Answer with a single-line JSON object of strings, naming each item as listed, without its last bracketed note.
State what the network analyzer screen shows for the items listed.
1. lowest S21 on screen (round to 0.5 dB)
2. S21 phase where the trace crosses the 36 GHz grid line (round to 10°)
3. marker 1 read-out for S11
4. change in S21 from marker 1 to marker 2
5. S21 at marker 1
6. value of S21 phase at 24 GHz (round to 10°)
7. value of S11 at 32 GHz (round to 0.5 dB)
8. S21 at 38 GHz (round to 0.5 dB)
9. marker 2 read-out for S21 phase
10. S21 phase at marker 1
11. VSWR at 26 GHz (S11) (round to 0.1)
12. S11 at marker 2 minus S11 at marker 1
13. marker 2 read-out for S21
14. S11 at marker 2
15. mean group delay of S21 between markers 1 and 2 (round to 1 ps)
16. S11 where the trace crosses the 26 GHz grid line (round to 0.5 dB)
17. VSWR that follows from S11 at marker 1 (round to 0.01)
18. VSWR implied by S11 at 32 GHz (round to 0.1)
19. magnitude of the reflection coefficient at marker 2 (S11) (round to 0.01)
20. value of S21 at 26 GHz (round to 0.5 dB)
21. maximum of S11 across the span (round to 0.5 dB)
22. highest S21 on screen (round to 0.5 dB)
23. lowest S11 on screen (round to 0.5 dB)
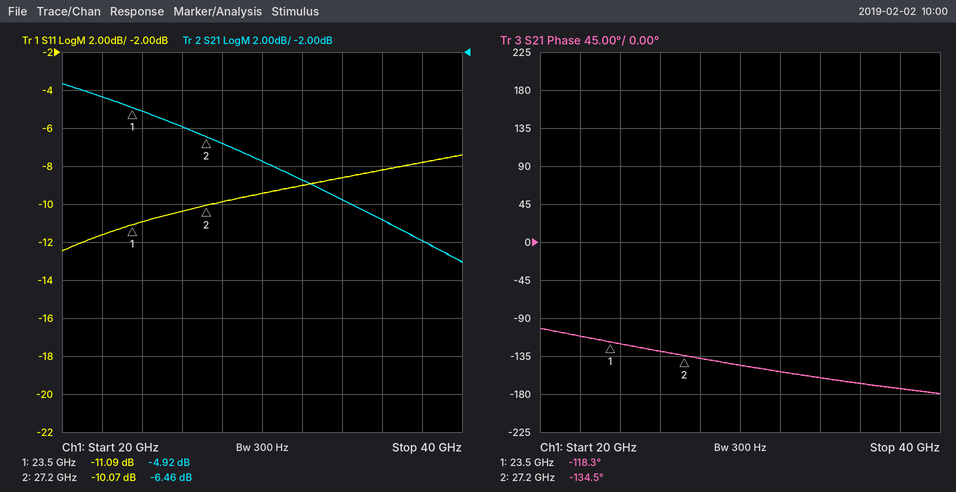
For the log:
{"lowest S21 on screen": "-13.0 dB", "S21 phase where the trace crosses the 36 GHz grid line": "-170°", "marker 1 read-out for S11": "-11.09 dB", "change in S21 from marker 1 to marker 2": "-1.54 dB", "S21 at marker 1": "-4.92 dB", "value of S21 phase at 24 GHz": "-120°", "value of S11 at 32 GHz": "-9.0 dB", "S21 at 38 GHz": "-12.0 dB", "marker 2 read-out for S21 phase": "-134.5°", "S21 phase at marker 1": "-118.3°", "VSWR at 26 GHz (S11)": "1.9", "S11 at marker 2 minus S11 at marker 1": "1.02 dB", "marker 2 read-out for S21": "-6.46 dB", "S11 at marker 2": "-10.07 dB", "mean group delay of S21 between markers 1 and 2": "12 ps", "S11 where the trace crosses the 26 GHz grid line": "-10.5 dB", "VSWR that follows from S11 at marker 1": "1.77", "VSWR implied by S11 at 32 GHz": "2.1", "magnitude of the reflection coefficient at marker 2 (S11)": "0.31", "value of S21 at 26 GHz": "-6.0 dB", "maximum of S11 across the span": "-7.5 dB", "highest S21 on screen": "-3.5 dB", "lowest S11 on screen": "-12.5 dB"}
